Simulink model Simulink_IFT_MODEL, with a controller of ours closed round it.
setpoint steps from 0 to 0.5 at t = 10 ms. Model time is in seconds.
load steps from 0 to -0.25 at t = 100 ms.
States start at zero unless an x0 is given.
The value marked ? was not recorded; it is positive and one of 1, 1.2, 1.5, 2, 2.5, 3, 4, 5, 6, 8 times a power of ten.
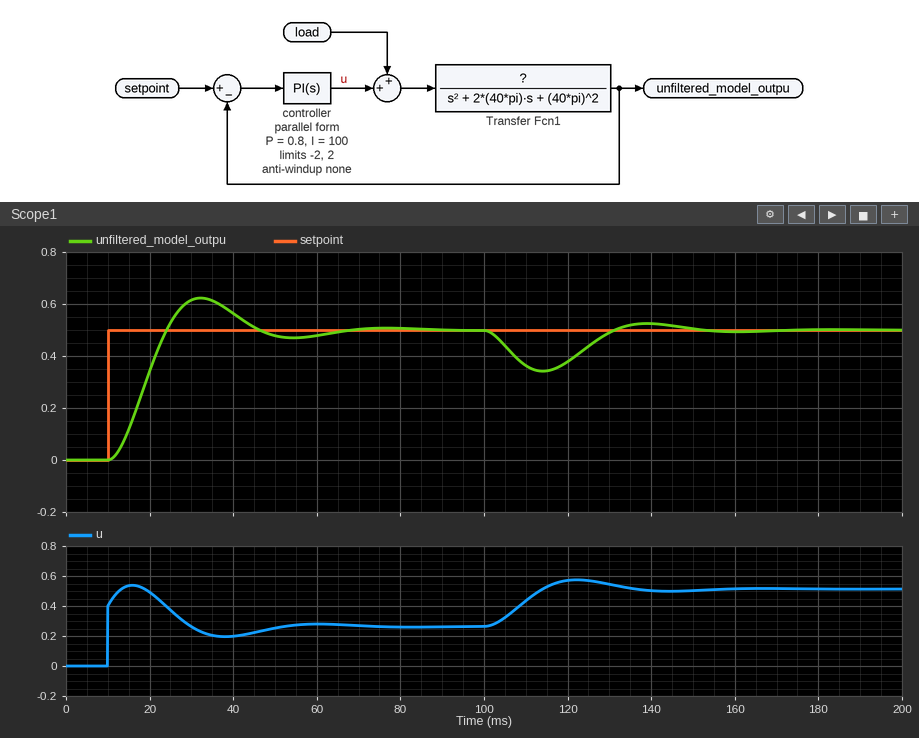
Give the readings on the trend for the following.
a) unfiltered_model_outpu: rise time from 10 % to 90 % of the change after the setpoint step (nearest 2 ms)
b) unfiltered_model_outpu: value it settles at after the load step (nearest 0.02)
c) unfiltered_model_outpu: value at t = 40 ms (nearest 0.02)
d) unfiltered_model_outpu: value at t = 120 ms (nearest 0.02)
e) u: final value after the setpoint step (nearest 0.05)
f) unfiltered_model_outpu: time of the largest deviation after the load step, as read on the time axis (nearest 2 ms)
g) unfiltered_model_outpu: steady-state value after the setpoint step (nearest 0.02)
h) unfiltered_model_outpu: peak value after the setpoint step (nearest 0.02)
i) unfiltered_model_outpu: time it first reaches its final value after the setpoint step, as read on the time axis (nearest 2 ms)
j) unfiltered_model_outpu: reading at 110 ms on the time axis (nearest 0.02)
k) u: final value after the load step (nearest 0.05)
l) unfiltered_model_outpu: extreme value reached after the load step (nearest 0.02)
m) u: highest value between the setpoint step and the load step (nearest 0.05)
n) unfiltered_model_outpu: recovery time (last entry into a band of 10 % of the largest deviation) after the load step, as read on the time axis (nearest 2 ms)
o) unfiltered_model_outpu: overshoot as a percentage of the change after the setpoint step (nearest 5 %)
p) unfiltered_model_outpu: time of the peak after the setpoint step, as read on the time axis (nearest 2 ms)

10 ms
0.50
0.56
0.38
0.25
114 ms
0.50
0.62
24 ms
0.36
0.50
0.34
0.55
146 ms
25 %
32 ms
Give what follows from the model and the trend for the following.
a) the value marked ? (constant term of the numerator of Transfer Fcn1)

30000
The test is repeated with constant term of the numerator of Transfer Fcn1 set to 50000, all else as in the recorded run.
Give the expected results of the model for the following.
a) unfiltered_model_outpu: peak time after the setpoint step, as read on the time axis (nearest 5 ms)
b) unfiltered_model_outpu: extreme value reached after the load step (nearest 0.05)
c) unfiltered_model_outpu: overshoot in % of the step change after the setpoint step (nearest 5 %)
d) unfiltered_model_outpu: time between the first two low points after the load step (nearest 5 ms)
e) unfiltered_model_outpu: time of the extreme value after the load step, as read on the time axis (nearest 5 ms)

25 ms
0.30
35 %
35 ms
110 ms
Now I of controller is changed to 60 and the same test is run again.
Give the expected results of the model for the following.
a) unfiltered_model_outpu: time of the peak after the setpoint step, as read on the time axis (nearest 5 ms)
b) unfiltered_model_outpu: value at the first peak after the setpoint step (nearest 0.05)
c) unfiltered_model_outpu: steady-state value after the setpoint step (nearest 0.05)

35 ms
0.55
0.50
